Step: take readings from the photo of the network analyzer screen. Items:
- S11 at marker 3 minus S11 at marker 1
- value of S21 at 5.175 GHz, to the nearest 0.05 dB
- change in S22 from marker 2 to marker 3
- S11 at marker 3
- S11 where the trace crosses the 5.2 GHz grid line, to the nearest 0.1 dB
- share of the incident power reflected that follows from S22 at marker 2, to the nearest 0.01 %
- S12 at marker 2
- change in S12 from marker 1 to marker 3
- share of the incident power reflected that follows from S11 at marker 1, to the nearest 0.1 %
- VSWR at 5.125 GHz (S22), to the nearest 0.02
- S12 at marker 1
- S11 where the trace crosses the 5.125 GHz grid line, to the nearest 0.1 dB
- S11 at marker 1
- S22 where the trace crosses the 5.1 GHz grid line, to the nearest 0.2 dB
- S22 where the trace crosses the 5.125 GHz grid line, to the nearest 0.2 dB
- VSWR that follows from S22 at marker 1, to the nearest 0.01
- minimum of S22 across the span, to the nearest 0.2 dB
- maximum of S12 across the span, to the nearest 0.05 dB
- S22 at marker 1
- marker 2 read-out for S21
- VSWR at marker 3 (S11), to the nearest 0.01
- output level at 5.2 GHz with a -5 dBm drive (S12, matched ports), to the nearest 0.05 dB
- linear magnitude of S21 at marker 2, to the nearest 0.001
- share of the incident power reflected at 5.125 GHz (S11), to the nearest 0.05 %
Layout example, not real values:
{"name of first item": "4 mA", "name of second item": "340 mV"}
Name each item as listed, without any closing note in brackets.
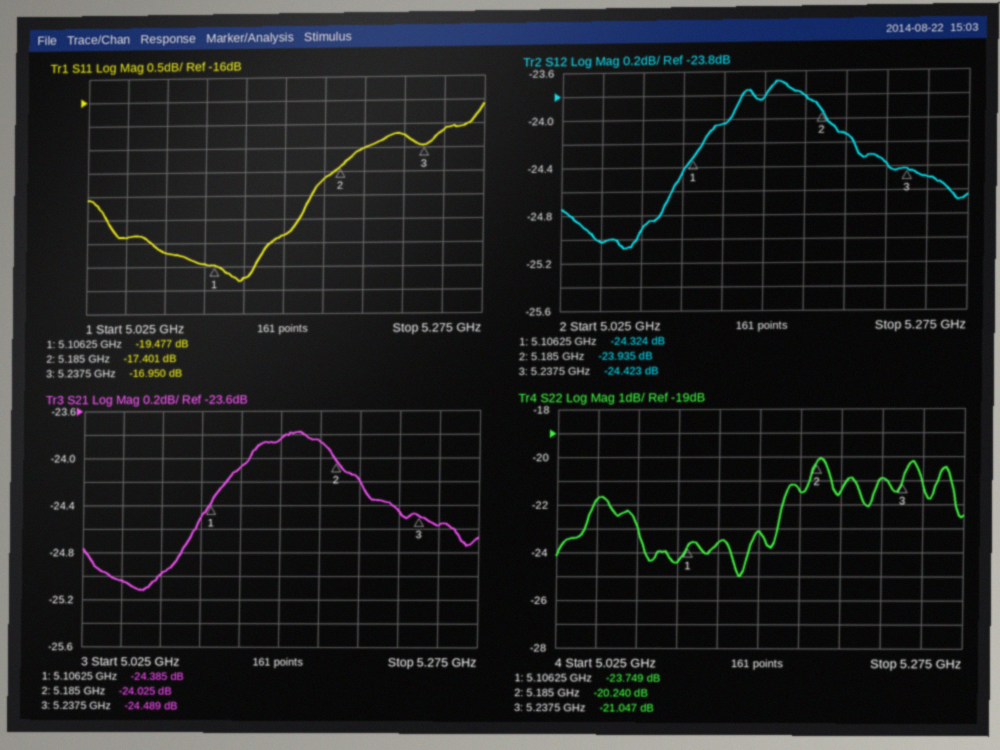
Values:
{"S11 at marker 3 minus S11 at marker 1": "2.527 dB", "value of S21 at 5.175 GHz, to the nearest 0.05 dB": "-23.85 dB", "change in S22 from marker 2 to marker 3": "-0.807 dB", "S11 at marker 3": "-16.950 dB", "S11 where the trace crosses the 5.2 GHz grid line, to the nearest 0.1 dB": "-17.0 dB", "share of the incident power reflected that follows from S22 at marker 2, to the nearest 0.01 %": "0.95 %", "S12 at marker 2": "-23.935 dB", "change in S12 from marker 1 to marker 3": "-0.099 dB", "share of the incident power reflected that follows from S11 at marker 1, to the nearest 0.1 %": "1.1 %", "VSWR at 5.125 GHz (S22), to the nearest 0.02": "1.14", "S12 at marker 1": "-24.324 dB", "S11 where the trace crosses the 5.125 GHz grid line, to the nearest 0.1 dB": "-19.7 dB", "S11 at marker 1": "-19.477 dB", "S22 where the trace crosses the 5.1 GHz grid line, to the nearest 0.2 dB": "-24.4 dB", "S22 where the trace crosses the 5.125 GHz grid line, to the nearest 0.2 dB": "-23.6 dB", "VSWR that follows from S22 at marker 1, to the nearest 0.01": "1.14", "minimum of S22 across the span, to the nearest 0.2 dB": "-25.0 dB", "maximum of S12 across the span, to the nearest 0.05 dB": "-23.70 dB", "S22 at marker 1": "-23.749 dB", "marker 2 read-out for S21": "-24.025 dB", "VSWR at marker 3 (S11), to the nearest 0.01": "1.33", "output level at 5.2 GHz with a -5 dBm drive (S12, matched ports), to the nearest 0.05 dB": "-29.15 dBm", "linear magnitude of S21 at marker 2, to the nearest 0.001": "0.063", "share of the incident power reflected at 5.125 GHz (S11), to the nearest 0.05 %": "1.05 %"}
